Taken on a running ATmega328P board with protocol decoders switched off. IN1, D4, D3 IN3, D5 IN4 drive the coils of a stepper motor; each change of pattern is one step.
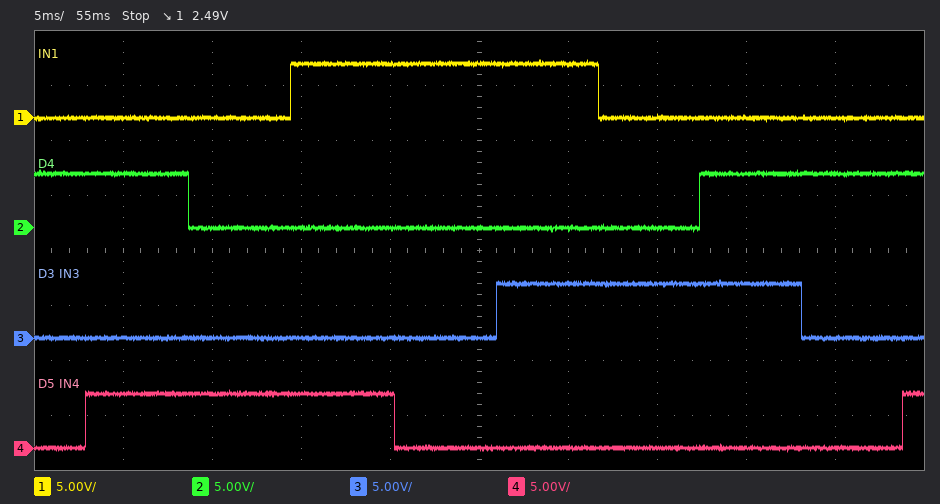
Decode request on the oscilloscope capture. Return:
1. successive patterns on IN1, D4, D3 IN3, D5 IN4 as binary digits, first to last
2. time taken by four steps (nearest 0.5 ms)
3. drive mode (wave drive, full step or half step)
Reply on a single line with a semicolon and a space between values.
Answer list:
0100 0101 0001 1001 1000 1010 0010 0110 0100 0101; 23.0 ms; half step
